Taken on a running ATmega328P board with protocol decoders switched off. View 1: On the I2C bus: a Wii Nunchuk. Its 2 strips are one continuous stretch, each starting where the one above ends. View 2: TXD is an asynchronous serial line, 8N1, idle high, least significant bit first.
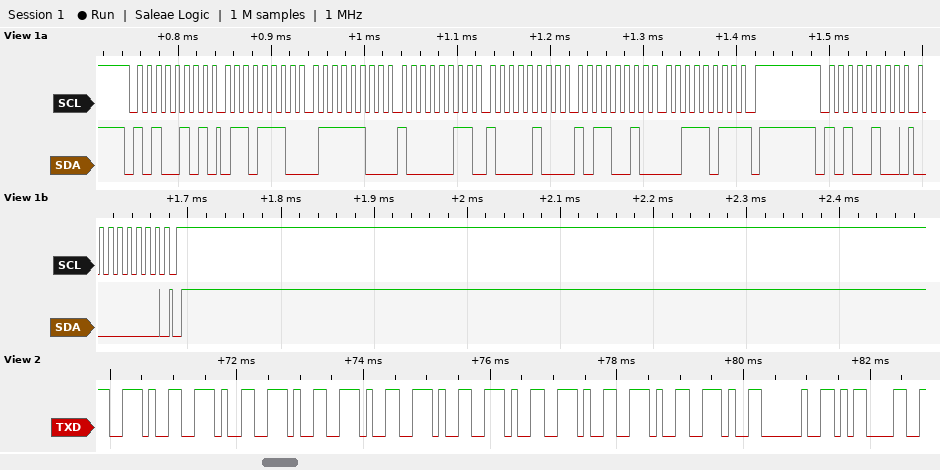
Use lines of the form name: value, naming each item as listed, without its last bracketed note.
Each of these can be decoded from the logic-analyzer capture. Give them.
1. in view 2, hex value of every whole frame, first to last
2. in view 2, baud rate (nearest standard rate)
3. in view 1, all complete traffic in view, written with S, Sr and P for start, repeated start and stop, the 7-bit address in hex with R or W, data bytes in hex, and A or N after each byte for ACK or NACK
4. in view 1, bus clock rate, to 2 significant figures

in view 2, hex value of every whole frame, first to last: 2E 2E 2E 2E 2E 2E 2E 2E 2E 20 0D
in view 2, baud rate: 9600 baud
in view 1, all complete traffic in view, written with S, Sr and P for start, repeated start and stop, the 7-bit address in hex with R or W, data bytes in hex, and A or N after each byte for ACK or NACK: S 52R A 6E A 7C A 83 A 84 A B2 A 3B N P S 52W A 00 A P
in view 1, bus clock rate, to 2 significant figures: 100 kHz
